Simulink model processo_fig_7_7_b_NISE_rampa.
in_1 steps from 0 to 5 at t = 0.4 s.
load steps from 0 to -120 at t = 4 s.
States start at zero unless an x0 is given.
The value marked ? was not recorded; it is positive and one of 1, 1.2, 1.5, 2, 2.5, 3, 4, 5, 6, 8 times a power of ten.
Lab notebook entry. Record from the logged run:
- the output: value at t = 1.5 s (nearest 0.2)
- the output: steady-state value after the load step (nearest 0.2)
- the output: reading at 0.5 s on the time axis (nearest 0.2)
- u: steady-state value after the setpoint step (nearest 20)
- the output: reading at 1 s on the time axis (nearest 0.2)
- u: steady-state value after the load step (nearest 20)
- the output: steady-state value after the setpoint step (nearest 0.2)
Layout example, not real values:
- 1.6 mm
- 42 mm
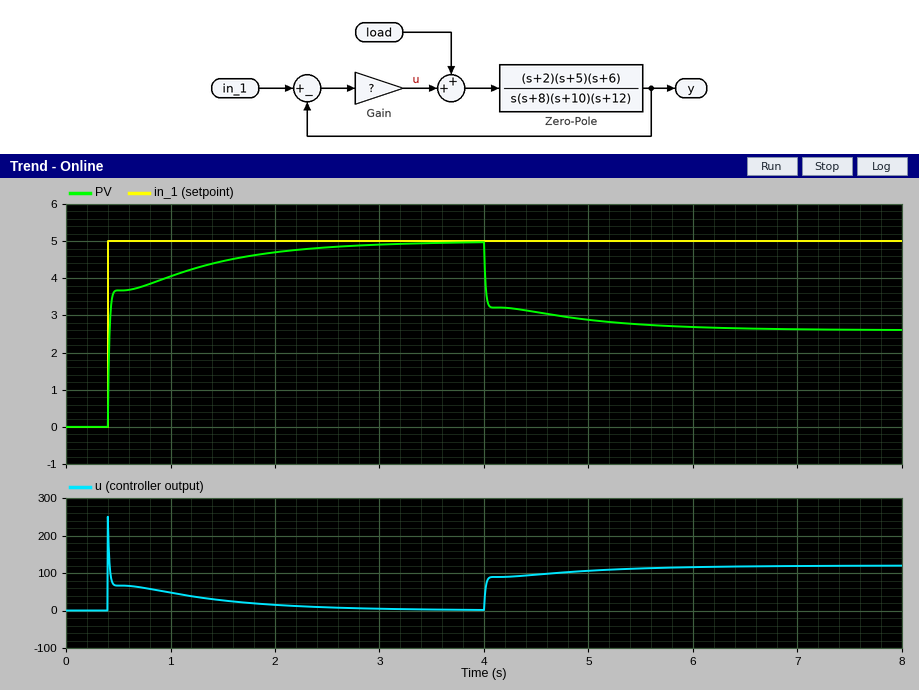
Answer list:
- 4.4
- 2.6
- 3.6
- 0
- 4.0
- 120
- 5.0
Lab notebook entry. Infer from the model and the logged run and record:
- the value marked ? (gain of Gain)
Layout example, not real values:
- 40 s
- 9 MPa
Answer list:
- 50
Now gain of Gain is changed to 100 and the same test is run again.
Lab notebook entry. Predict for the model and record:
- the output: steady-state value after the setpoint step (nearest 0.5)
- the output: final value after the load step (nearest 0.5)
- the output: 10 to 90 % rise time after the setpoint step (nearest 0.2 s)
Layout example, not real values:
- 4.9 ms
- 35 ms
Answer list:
- 5.0
- 4.0
- 0.6 s
